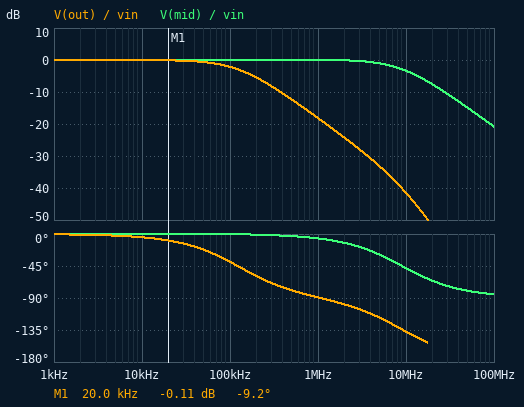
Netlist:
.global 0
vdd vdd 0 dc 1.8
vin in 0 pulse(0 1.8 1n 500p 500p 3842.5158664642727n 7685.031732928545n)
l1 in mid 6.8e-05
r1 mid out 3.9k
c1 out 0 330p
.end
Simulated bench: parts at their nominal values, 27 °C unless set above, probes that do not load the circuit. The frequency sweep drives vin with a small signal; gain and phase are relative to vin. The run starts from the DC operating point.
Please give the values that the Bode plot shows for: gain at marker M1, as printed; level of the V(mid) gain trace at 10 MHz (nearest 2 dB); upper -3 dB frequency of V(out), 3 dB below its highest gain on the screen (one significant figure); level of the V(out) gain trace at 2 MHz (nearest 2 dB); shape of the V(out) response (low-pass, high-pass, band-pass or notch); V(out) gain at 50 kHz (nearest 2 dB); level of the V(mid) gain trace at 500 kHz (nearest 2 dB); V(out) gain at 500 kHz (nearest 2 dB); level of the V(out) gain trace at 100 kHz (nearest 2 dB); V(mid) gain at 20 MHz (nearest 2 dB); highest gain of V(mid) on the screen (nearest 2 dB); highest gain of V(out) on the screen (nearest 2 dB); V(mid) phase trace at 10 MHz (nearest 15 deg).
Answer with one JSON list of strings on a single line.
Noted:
["-0.11 dB", "-4 dB", "100 kHz", "-24 dB", "low-pass", "0 dB", "0 dB", "-12 dB", "-2 dB", "-8 dB", "0 dB", "0 dB", "-45 deg"]
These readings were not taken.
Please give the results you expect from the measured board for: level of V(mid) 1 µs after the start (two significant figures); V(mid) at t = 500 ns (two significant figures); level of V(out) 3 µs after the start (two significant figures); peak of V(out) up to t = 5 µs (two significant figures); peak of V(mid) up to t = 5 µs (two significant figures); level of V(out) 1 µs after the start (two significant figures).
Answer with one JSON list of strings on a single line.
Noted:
["1.8 V", "1.8 V", "1.6 V", "1.7 V", "1.8 V", "970 mV"]
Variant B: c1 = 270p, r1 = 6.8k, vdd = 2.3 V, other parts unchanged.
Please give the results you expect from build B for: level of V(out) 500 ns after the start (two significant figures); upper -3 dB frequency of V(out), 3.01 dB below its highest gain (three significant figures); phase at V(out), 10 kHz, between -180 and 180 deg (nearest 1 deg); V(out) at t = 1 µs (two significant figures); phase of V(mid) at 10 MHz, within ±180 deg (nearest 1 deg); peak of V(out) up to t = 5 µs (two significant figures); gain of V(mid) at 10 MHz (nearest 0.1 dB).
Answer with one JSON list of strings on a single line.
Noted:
["420 mV", "87.2 kHz", "-7 deg", "750 mV", "-32 deg", "1.6 V", "-1.4 dB"]
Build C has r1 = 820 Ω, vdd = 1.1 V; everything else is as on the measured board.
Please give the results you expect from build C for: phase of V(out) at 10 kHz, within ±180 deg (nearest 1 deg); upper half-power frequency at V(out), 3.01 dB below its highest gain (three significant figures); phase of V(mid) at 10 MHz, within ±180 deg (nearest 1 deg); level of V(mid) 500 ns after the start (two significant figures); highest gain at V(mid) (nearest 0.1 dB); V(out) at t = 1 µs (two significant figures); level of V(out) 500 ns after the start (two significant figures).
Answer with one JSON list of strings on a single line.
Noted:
["-1 deg", "789 kHz", "-82 deg", "2.0 V", "1.5 dB", "1.8 V", "1.6 V"]
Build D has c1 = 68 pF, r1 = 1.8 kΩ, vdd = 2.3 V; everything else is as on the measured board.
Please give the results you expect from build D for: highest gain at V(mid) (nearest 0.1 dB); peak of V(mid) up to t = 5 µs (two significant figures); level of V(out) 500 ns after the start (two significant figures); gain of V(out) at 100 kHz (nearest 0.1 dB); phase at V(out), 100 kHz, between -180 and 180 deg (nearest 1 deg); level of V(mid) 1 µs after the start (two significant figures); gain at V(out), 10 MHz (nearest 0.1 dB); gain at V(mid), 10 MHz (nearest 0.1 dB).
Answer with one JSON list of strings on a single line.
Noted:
["1.5 dB", "2.1 V", "1.8 V", "0 dB", "-4 deg", "1.8 V", "-25.5 dB", "-7.7 dB"]
